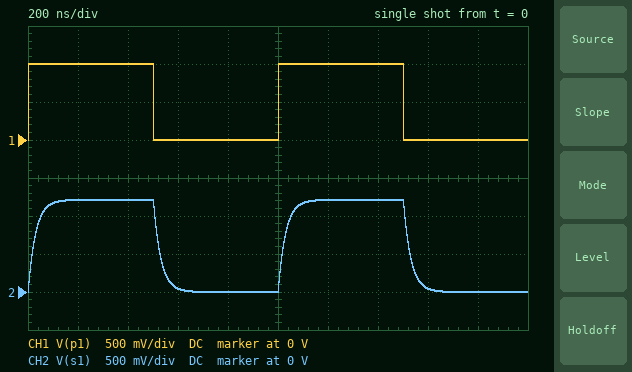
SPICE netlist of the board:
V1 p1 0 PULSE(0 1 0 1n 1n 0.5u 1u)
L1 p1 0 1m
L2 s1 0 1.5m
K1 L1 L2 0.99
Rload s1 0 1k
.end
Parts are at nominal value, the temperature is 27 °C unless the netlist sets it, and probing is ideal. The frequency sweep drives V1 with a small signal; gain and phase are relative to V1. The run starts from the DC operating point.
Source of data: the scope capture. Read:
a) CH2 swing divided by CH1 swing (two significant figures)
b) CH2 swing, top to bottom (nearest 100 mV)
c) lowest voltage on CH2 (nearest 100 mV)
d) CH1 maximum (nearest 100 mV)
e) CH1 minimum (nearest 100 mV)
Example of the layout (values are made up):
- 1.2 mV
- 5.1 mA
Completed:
- 1.2
- 1.2 V
- 0 V
- 1.0 V
- 0 V
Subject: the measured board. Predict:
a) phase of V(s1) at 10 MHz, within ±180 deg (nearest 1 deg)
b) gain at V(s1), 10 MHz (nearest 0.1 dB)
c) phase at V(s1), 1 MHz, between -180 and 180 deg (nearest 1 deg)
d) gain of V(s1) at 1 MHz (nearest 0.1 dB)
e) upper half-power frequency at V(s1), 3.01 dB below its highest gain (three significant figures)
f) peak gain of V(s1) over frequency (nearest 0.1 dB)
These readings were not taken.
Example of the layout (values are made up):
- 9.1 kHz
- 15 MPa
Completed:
- -62 deg
- -4.9 dB
- -11 deg
- 1.5 dB
- 5.33 MHz
- 1.7 dB
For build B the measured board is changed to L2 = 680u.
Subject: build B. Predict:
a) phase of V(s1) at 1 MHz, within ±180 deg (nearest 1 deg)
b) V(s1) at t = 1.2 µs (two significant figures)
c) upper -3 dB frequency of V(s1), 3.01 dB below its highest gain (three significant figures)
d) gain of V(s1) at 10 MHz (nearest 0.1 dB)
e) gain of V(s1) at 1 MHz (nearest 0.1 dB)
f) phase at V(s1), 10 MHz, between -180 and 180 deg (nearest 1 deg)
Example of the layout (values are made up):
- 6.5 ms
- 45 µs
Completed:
- -5 deg
- 820 mV
- 11.8 MHz
- -4.1 dB
- -1.8 dB
- -40 deg
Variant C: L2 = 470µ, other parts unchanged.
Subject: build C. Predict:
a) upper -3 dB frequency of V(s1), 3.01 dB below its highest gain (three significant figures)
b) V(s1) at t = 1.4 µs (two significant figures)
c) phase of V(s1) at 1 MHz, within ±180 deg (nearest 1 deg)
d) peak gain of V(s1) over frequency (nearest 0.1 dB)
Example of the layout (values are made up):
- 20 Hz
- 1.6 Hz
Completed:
- 17.0 MHz
- 680 mV
- -3 deg
- -3.4 dB
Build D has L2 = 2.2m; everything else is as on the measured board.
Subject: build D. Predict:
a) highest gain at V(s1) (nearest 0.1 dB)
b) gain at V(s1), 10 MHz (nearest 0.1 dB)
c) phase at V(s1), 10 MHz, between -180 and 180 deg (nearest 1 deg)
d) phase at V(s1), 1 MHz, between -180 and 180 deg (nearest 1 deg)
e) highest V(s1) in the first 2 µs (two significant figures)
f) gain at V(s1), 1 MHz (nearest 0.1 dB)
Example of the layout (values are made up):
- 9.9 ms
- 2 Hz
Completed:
- 3.3 dB
- -6.0 dB
- -70 deg
- -15 deg
- 1.5 V
- 3.0 dB
